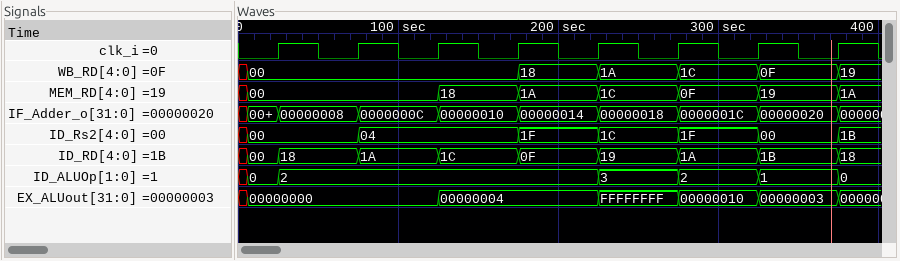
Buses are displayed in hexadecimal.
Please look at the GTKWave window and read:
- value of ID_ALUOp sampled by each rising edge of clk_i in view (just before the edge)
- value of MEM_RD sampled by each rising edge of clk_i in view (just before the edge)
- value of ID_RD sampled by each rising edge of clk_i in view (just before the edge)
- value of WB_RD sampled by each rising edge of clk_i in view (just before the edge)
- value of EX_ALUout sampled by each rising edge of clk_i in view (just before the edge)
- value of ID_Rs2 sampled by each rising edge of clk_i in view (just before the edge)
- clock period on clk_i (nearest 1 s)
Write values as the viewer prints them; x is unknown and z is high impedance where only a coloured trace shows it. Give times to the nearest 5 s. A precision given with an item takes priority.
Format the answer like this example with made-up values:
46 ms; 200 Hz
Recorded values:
0, 2, 2, 2, 2, 3, 2, 1; 00, 00, 00, 18, 1A, 1C, 0F, 19; 00, 18, 1A, 1C, 0F, 19, 1A, 1B; 00, 00, 00, 00, 18, 1A, 1C, 0F; 00000000, 00000000, 00000000, 00000004, 00000004, FFFFFFFF, 00000010, 00000003; 00, 00, 04, 04, 1F, 1C, 1F, 00; 50 s
